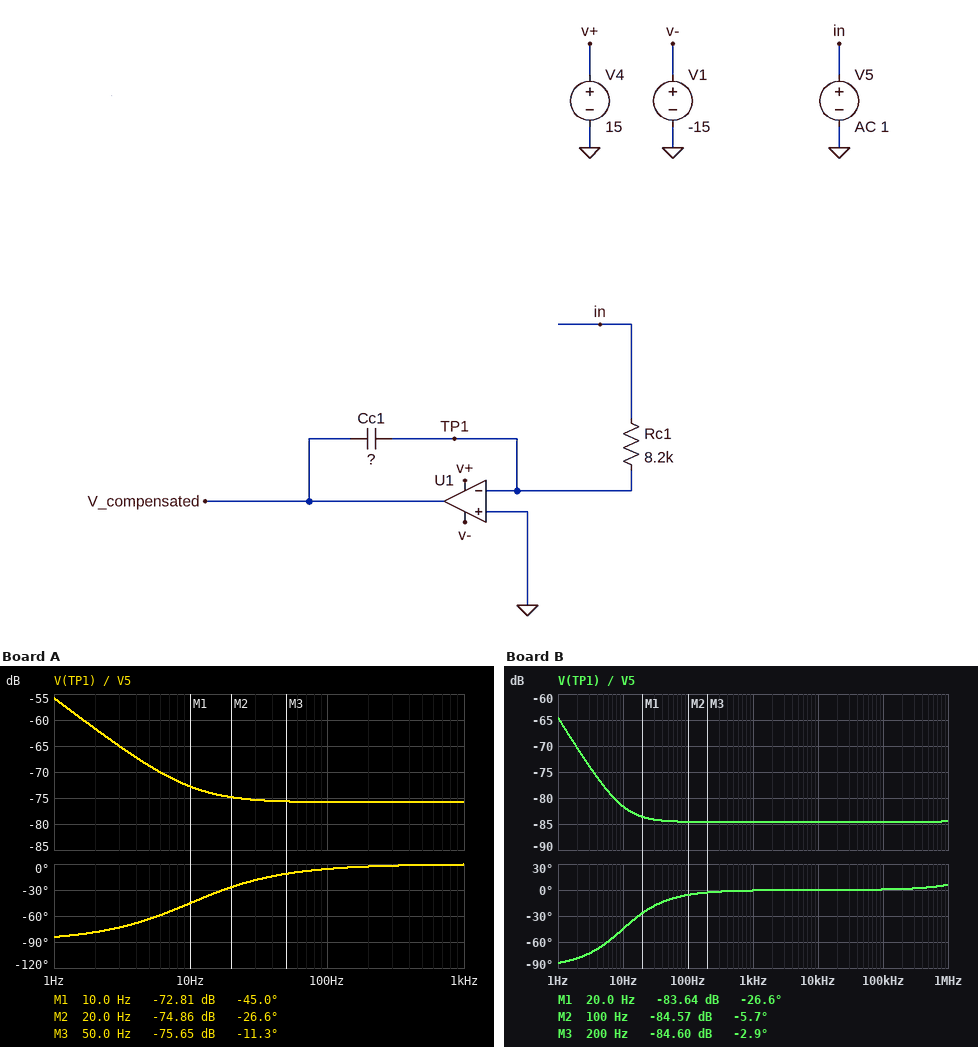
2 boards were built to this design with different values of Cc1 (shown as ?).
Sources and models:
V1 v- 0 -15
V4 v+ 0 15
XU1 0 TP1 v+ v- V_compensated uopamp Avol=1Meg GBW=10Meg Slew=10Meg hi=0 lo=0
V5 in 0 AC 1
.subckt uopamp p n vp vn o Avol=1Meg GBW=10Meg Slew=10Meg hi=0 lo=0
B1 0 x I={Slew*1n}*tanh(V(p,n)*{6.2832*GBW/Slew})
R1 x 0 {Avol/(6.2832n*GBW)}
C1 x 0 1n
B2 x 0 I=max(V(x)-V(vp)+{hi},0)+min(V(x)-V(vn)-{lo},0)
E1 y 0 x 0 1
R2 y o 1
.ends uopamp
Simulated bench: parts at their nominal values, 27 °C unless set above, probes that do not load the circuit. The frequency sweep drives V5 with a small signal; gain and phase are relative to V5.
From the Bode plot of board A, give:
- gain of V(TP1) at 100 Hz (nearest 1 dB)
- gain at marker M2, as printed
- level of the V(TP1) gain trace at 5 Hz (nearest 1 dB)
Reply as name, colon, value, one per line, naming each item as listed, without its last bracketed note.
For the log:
gain of V(TP1) at 100 Hz: -76 dB
gain at marker M2, as printed: -74.86 dB
level of the V(TP1) gain trace at 5 Hz: -69 dB
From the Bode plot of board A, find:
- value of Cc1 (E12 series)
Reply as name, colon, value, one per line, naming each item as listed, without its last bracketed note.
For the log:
value of Cc1: 12 nF
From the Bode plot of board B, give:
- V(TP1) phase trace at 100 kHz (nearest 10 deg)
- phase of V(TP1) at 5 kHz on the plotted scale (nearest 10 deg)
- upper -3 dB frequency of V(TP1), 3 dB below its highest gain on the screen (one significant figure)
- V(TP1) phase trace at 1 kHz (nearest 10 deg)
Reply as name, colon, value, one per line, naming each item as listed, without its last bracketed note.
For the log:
V(TP1) phase trace at 100 kHz: 0 deg
phase of V(TP1) at 5 kHz on the plotted scale: 0 deg
upper -3 dB frequency of V(TP1), 3 dB below its highest gain on the screen: 1 Hz
V(TP1) phase trace at 1 kHz: 0 deg
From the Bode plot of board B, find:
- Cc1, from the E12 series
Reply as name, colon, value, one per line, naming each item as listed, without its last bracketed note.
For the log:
Cc1, from the E12 series: 33 nF
